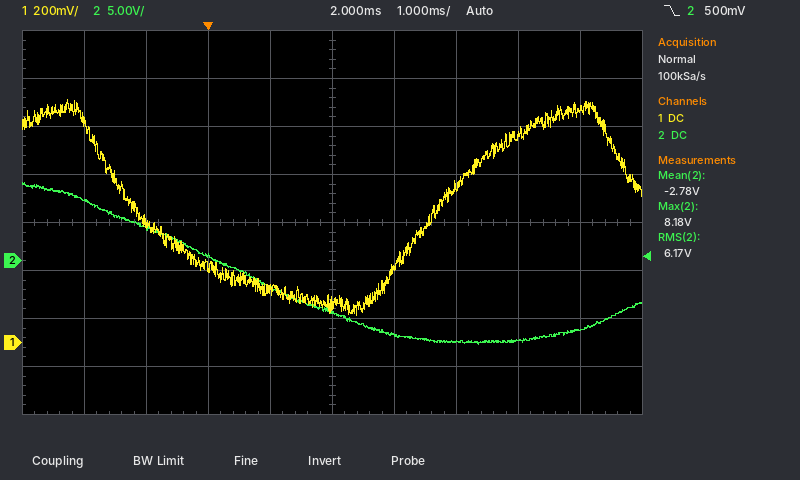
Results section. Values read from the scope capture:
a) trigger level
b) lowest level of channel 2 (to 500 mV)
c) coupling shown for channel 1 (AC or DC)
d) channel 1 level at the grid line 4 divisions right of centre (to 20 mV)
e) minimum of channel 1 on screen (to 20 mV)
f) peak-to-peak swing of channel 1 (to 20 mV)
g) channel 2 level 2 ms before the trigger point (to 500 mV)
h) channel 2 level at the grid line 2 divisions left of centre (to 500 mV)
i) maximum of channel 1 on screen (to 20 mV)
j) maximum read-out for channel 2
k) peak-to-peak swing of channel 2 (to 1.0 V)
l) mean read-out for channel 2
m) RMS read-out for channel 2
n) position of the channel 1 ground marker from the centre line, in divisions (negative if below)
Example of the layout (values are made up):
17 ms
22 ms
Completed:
500 mV
-8.5 V
DC
980 mV
120 mV
900 mV
6.5 V
500 mV
1.02 V
8.18 V
17.0 V
-2.78 V
6.17 V
-2.5 div
